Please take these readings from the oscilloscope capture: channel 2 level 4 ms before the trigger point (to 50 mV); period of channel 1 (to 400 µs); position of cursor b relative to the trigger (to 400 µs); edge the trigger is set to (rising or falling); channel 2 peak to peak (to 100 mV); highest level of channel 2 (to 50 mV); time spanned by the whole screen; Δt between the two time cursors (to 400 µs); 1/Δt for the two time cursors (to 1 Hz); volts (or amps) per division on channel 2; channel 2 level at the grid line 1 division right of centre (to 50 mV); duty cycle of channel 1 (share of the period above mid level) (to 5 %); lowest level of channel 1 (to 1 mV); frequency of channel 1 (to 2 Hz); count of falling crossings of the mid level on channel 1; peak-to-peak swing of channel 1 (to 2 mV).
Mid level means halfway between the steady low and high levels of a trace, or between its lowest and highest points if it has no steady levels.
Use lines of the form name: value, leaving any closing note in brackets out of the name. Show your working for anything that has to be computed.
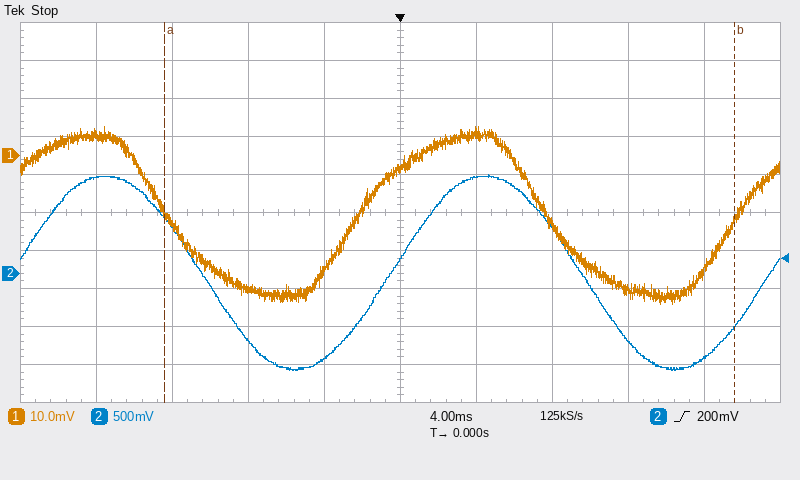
channel 2 level 4 ms before the trigger point: -1.10 V
period of channel 1: 20.0 ms
position of cursor b relative to the trigger: +17.6 ms
edge the trigger is set to: rising
channel 2 peak to peak: 2.60 V
highest level of channel 2: 1.30 V
time spanned by the whole screen: 40 ms
Δt between the two time cursors: 30.0 ms
1/Δt for the two time cursors: 1 / 30.0 ms ≈ 33 Hz
volts (or amps) per division on channel 2: 500 mV
channel 2 level at the grid line 1 division right of centre: 1.25 V
duty cycle of channel 1 (share of the period above mid level): 50 %
lowest level of channel 1: -39 mV
frequency of channel 1: 1 / 20.0 ms ≈ 50 Hz
count of falling crossings of the mid level on channel 1: 2
peak-to-peak swing of channel 1: 46 mV
